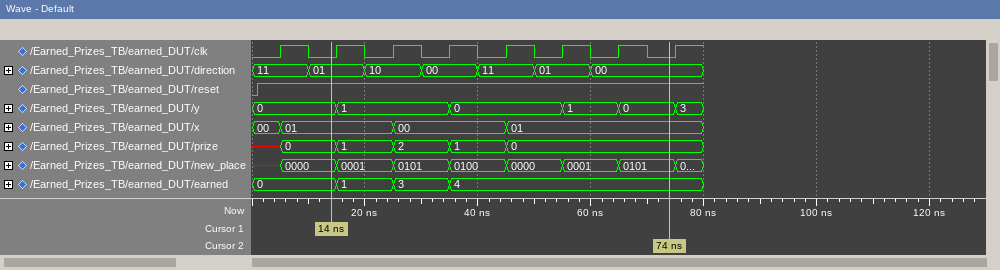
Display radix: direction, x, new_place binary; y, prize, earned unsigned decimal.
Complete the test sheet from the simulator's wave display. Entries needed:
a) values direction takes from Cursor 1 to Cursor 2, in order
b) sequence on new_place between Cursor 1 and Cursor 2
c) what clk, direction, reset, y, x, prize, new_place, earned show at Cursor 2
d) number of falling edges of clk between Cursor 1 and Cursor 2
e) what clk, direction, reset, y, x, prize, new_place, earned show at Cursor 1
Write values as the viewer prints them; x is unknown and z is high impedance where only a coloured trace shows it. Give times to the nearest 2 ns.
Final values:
01, 10, 00, 11, 01, 00
0000, 0001, 0101, 0100, 0000, 0001, 0101
clk=0, direction=00, reset=1, y=0, x=01, prize=0, new_place=0101, earned=4
6
clk=0, direction=01, reset=1, y=0, x=01, prize=0, new_place=0000, earned=0
